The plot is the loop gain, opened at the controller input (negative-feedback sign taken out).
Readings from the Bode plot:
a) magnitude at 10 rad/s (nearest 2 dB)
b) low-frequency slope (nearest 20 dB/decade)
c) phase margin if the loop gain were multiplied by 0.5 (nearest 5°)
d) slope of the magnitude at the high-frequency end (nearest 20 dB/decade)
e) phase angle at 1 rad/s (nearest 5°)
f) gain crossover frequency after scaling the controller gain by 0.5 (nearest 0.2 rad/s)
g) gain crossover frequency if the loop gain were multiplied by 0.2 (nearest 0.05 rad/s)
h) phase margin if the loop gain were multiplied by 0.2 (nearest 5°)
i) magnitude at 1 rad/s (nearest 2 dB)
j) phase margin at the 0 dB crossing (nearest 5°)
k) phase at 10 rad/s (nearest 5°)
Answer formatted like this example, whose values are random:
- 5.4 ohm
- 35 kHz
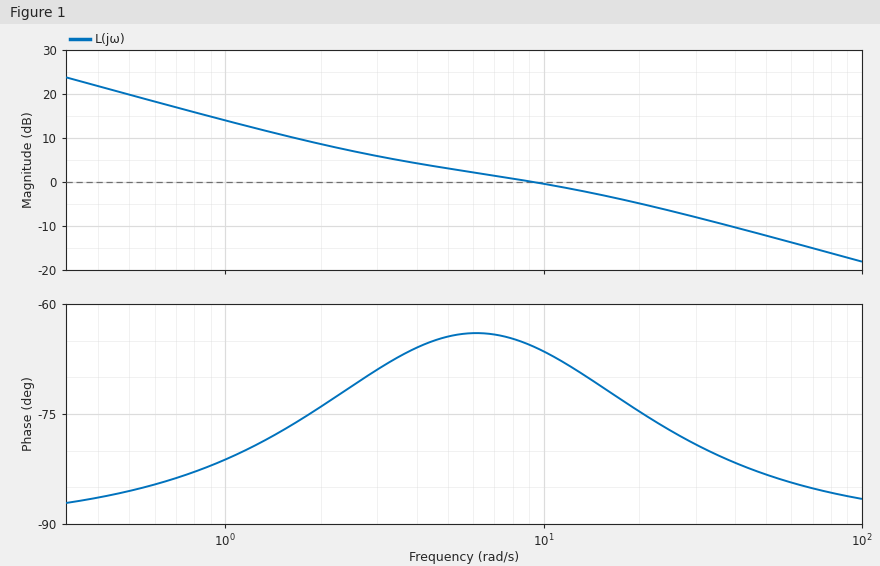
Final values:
- 0 dB
- -20 dB/decade
- 110°
- -20 dB/decade
- -80°
- 3.0 rad/s
- 1.00 rad/s
- 100°
- 14 dB
- 115°
- -65°
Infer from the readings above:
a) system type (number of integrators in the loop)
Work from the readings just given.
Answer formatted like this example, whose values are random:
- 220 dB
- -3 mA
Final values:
- 1
